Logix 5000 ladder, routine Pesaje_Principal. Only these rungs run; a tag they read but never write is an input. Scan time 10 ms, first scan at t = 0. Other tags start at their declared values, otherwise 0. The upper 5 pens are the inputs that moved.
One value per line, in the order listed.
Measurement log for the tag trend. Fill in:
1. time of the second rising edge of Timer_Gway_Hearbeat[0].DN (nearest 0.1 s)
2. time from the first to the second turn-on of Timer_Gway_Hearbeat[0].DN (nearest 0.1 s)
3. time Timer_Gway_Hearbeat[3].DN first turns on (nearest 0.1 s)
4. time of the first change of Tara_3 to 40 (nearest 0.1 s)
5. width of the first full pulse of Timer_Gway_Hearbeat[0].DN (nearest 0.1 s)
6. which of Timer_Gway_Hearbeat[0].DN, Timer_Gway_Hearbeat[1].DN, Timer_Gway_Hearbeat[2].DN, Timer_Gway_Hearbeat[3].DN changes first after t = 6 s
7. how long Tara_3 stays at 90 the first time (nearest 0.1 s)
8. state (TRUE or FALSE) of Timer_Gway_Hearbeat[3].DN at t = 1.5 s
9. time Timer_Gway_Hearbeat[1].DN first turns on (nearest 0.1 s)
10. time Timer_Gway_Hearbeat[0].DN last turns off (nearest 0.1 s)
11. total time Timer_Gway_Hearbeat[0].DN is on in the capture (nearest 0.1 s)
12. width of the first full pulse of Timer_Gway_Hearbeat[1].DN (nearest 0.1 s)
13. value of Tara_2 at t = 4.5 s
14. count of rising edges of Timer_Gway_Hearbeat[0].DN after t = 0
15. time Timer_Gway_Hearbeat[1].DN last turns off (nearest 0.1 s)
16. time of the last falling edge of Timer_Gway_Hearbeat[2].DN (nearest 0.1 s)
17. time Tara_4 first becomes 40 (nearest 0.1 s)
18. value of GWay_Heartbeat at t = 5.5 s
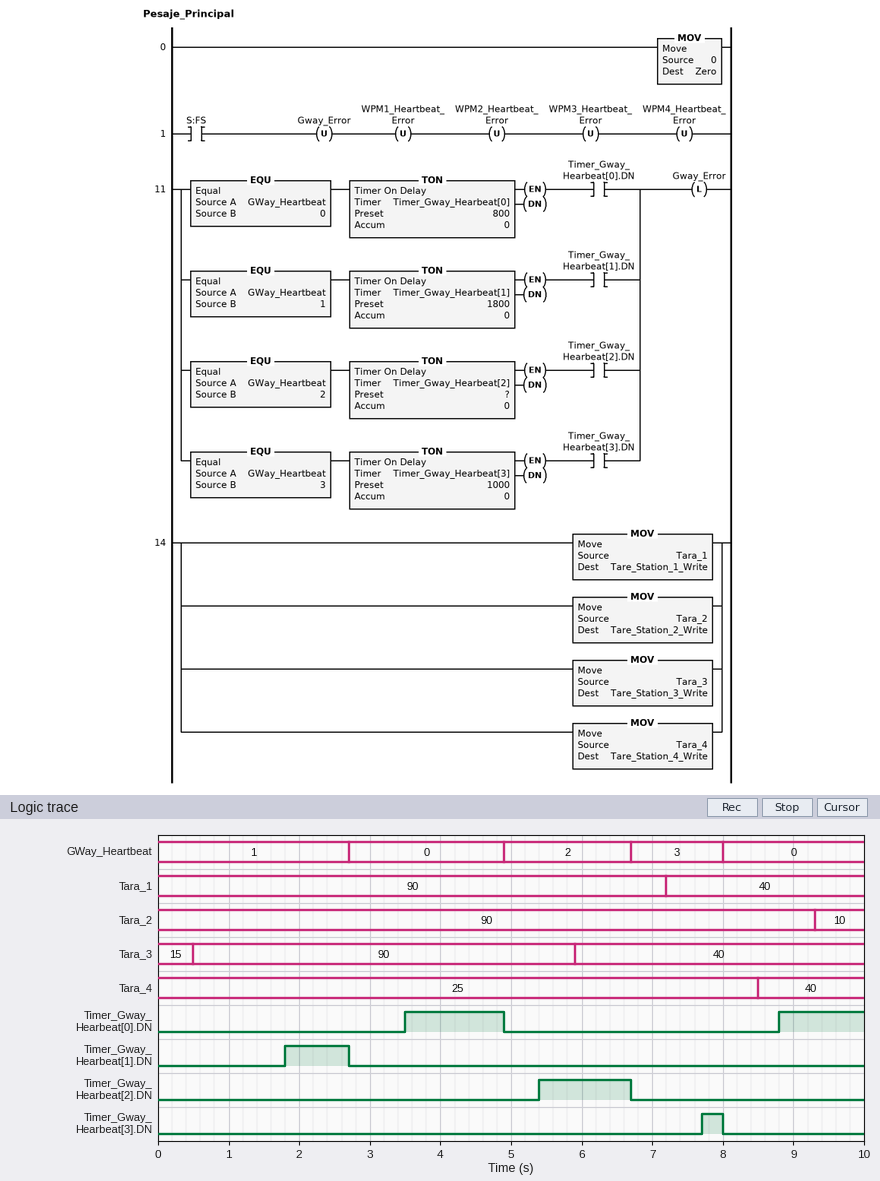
8.8 s
5.3 s
7.7 s
5.9 s
1.4 s
Timer_Gway_Hearbeat[2].DN
5.4 s
FALSE
1.8 s
4.9 s
2.6 s
0.9 s
90
2
2.7 s
6.7 s
8.5 s
2
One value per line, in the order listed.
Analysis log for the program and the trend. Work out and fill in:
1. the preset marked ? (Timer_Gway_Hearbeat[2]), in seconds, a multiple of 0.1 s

0.5 s
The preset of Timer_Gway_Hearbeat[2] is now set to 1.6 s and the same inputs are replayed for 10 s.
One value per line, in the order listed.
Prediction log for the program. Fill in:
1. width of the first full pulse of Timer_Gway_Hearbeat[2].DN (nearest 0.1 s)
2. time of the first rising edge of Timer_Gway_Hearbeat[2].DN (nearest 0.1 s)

0.2 s
6.5 s
